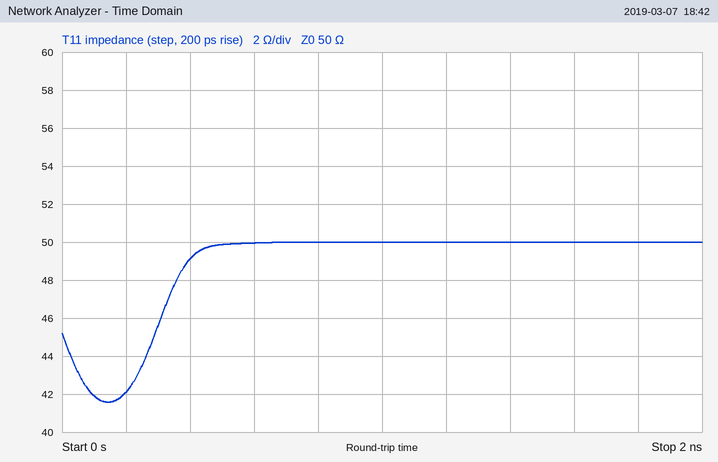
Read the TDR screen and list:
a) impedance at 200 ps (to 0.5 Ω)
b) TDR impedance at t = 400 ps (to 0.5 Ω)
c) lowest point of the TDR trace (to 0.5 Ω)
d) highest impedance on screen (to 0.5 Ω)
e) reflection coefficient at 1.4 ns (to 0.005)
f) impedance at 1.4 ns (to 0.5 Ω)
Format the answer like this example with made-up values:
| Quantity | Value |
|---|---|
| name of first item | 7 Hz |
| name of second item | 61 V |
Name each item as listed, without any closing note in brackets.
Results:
| Quantity | Value |
|---|---|
| impedance at 200 ps | 42.0 Ω |
| TDR impedance at t = 400 ps | 49.0 Ω |
| lowest point of the TDR trace | 41.5 Ω |
| highest impedance on screen | 50.0 Ω |
| reflection coefficient at 1.4 ns | 0.000 |
| impedance at 1.4 ns | 50.0 Ω |
